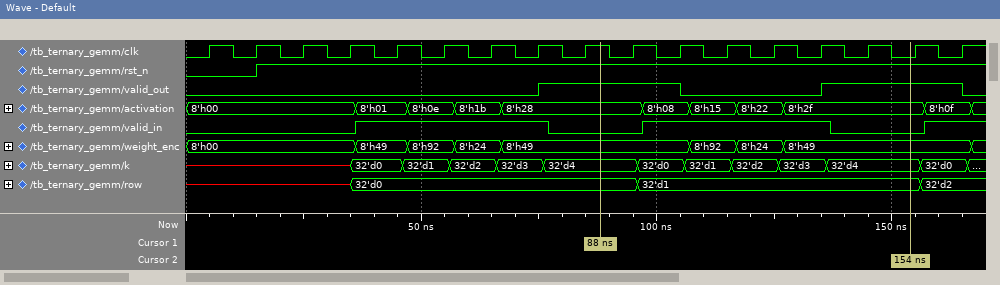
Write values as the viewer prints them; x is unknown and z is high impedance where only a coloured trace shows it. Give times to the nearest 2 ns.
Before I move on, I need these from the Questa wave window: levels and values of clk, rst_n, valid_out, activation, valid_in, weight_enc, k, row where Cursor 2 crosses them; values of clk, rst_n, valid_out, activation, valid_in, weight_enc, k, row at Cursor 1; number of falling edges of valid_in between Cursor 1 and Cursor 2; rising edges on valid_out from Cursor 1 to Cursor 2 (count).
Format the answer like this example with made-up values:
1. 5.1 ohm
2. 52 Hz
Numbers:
1. clk=0, rst_n=1, valid_out=1, activation=8'h2f, valid_in=0, weight_enc=8'h49, k=32'd4, row=32'd1
2. clk=1, rst_n=1, valid_out=1, activation=8'h28, valid_in=0, weight_enc=8'h49, k=32'd4, row=32'd0
3. 1
4. 1
